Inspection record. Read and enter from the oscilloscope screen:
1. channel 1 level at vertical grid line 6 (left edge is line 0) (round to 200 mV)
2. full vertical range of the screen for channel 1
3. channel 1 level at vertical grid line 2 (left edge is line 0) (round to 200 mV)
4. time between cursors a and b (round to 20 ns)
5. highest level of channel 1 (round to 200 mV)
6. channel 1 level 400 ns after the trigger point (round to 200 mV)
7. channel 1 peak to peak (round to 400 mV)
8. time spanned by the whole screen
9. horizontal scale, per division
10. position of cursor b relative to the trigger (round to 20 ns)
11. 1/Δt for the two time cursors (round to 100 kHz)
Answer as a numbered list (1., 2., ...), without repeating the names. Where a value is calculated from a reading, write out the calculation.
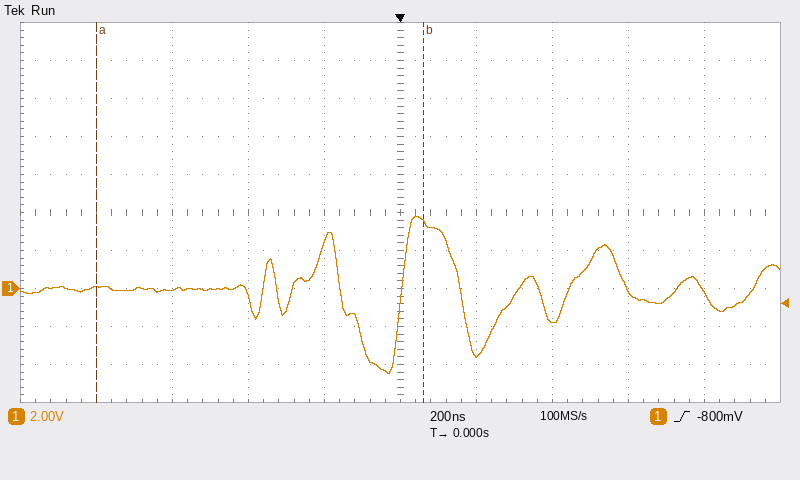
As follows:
1. -3.4 V
2. 20 V
3. 0.0 V
4. 860 ns
5. 3.8 V
6. -1.8 V
7. 8.4 V
8. 2 µs
9. 200 ns
10. +60 ns
11. 1 / 860 ns ≈ 1.2 MHz
